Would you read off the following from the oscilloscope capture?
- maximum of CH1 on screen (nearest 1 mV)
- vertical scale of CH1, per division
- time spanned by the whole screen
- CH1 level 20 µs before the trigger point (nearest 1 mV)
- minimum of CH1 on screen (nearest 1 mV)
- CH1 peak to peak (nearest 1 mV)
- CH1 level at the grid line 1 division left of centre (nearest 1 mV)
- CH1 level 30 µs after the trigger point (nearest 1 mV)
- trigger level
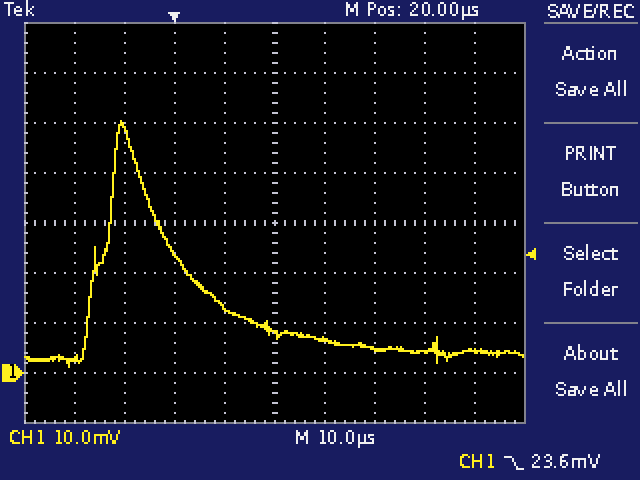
50 mV
10 mV
100 µs
3 mV
1 mV
49 mV
13 mV
7 mV
23.6 mV
